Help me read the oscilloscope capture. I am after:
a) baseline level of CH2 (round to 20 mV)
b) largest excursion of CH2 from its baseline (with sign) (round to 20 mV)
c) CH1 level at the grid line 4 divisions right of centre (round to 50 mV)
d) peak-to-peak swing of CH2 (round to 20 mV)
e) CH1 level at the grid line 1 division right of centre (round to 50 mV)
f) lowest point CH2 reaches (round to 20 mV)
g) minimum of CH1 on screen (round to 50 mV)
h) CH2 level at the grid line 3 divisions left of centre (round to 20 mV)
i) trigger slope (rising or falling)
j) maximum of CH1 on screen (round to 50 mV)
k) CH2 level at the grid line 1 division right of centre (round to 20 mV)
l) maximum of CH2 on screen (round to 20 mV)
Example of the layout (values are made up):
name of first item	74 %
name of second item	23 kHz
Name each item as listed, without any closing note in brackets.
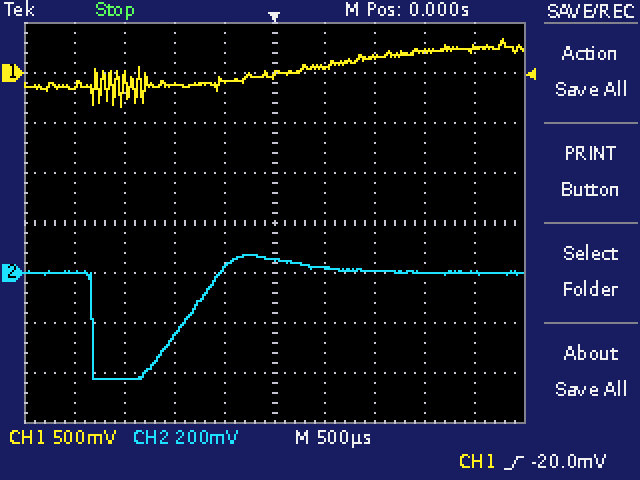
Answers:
baseline level of CH2	0 mV
largest excursion of CH2 from its baseline (with sign)	-420 mV
CH1 level at the grid line 4 divisions right of centre	250 mV
peak-to-peak swing of CH2	500 mV
CH1 level at the grid line 1 division right of centre	50 mV
lowest point CH2 reaches	-420 mV
minimum of CH1 on screen	-350 mV
CH2 level at the grid line 3 divisions left of centre	-420 mV
trigger slope	rising
maximum of CH1 on screen	350 mV
CH2 level at the grid line 1 division right of centre	20 mV
maximum of CH2 on screen	80 mV
